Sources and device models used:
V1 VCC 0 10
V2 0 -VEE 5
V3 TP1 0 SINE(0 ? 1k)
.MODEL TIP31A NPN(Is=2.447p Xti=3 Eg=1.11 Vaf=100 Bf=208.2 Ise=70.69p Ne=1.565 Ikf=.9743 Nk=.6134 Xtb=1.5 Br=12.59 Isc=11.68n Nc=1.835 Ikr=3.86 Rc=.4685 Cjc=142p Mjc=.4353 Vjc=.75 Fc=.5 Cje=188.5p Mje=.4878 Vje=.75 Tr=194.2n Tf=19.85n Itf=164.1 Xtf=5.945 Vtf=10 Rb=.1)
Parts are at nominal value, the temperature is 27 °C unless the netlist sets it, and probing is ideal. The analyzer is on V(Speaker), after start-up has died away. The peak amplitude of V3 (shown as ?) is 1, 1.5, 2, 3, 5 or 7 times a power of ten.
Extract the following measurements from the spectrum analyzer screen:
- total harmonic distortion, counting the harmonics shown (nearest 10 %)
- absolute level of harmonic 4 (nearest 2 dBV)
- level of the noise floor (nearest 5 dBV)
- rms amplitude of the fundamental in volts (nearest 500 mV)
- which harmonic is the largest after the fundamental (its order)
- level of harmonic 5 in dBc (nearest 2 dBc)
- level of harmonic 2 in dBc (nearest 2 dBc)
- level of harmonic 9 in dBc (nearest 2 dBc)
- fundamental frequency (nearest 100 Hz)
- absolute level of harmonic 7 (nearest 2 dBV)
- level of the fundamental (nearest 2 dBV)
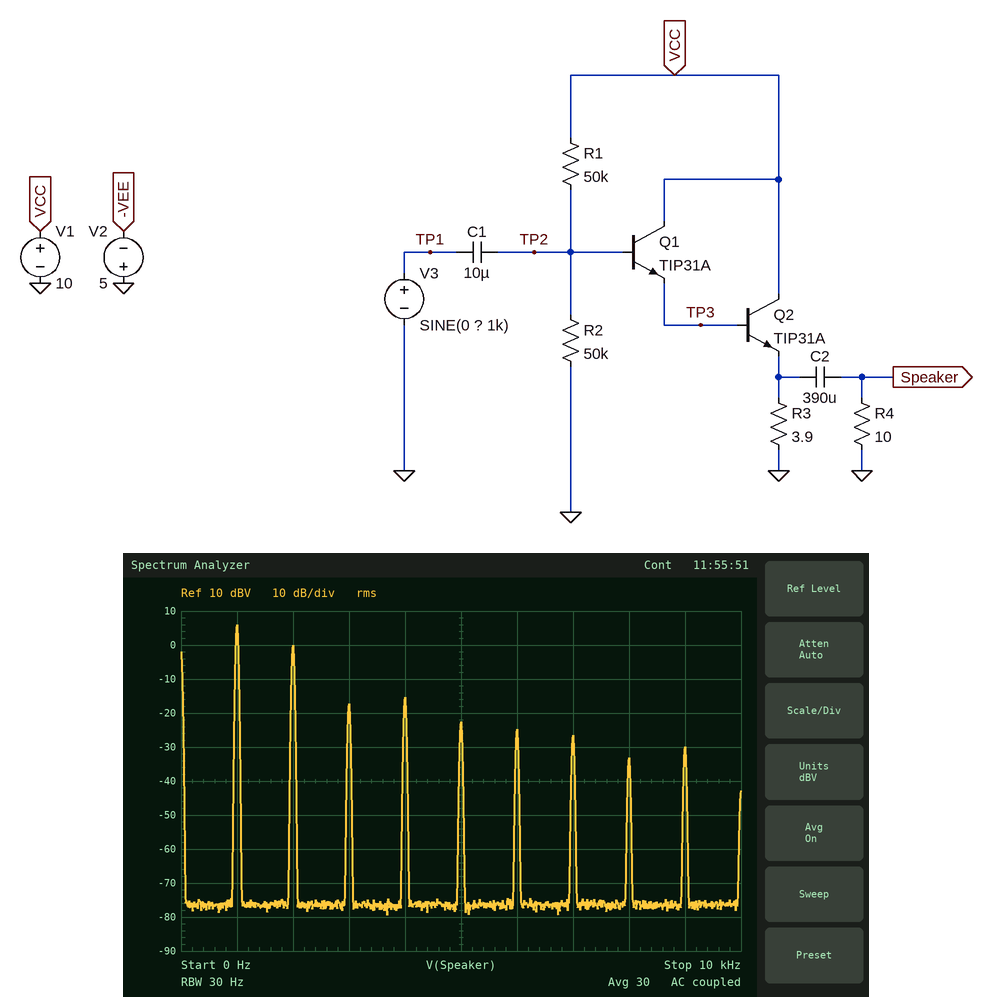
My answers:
50 %
-16 dBV
-75 dBV
2.0 V
2
-28 dBc
-6 dBc
-36 dBc
1.0 kHz
-26 dBV
6 dBV
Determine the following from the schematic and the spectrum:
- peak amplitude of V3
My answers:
7 V
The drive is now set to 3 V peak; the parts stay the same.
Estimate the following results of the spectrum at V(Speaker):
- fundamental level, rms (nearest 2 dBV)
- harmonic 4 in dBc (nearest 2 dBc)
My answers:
2 dBV
-32 dBc
